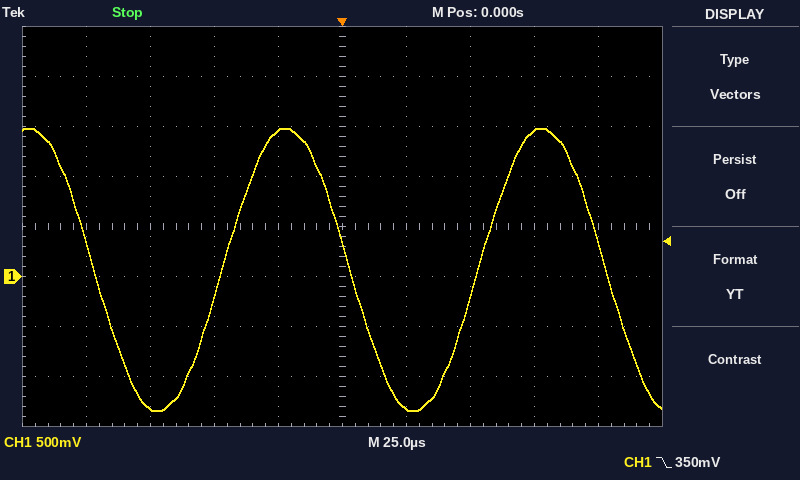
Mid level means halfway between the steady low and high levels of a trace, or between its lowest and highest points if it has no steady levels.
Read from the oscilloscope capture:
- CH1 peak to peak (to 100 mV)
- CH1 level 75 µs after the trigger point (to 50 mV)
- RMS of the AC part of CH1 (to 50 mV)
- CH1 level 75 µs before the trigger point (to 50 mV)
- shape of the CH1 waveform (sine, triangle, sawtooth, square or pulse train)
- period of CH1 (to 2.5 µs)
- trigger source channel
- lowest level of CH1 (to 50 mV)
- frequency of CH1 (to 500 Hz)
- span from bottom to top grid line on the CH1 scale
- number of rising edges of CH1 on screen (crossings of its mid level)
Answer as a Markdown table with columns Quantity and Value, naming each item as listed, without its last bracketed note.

| Quantity | Value |
|---|---|
| CH1 peak to peak | 2.80 V |
| CH1 level 75 µs after the trigger point | 1.45 V |
| RMS of the AC part of CH1 | 1.00 V |
| CH1 level 75 µs before the trigger point | -1.30 V |
| shape of the CH1 waveform | sine |
| period of CH1 | 100.0 µs |
| trigger source channel | CH1 |
| lowest level of CH1 | -1.35 V |
| frequency of CH1 | 10.0 kHz |
| span from bottom to top grid line on the CH1 scale | 4 V |
| number of rising edges of CH1 on screen | 2 |
